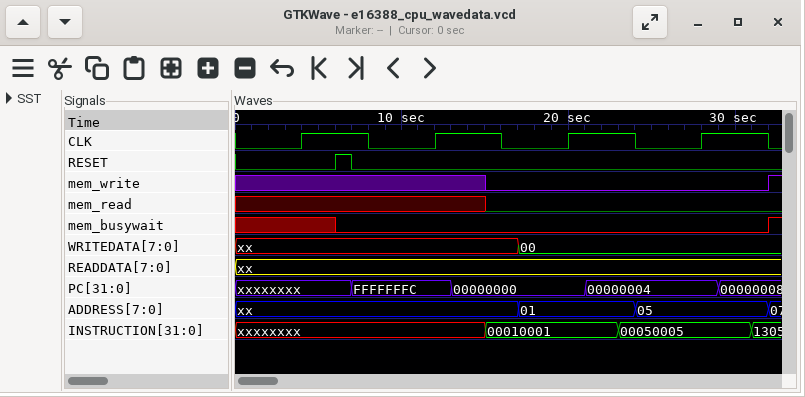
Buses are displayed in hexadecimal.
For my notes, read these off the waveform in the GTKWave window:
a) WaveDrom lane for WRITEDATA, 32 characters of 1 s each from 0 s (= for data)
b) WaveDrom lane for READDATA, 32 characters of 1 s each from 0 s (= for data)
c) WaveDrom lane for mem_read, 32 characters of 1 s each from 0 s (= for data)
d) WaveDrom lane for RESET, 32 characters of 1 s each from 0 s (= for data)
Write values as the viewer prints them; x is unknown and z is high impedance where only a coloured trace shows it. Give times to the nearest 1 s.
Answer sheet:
{name: 'WRITEDATA', wave: 'x................=..............', data: '00'}
{name: 'READDATA', wave: 'x...............................'}
{name: 'mem_read', wave: 'x..............0................'}
{name: 'RESET', wave: '0.....10........................'}
